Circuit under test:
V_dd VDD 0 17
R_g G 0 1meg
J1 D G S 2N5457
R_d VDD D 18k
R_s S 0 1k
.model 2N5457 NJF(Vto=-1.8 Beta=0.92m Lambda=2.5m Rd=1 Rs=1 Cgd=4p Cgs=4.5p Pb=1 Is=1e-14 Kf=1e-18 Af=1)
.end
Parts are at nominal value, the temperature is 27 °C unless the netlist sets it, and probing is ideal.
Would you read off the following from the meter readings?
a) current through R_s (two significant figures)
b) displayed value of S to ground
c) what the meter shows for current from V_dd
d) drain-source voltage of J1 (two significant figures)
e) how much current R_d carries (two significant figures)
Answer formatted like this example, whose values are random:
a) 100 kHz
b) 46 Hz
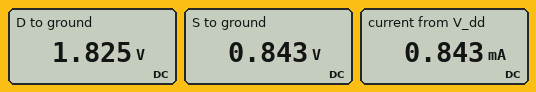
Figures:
a) 840 µA
b) 0.843 V
c) 0.843 mA
d) 980 mV
e) 840 µA
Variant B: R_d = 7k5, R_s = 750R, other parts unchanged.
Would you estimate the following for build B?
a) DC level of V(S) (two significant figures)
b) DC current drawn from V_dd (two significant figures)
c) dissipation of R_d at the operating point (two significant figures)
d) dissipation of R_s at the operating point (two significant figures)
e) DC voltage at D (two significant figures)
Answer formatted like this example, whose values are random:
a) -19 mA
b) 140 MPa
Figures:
a) 760 mV
b) 1.0 mA
c) 7.7 mW
d) 770 µW
e) 9.4 V
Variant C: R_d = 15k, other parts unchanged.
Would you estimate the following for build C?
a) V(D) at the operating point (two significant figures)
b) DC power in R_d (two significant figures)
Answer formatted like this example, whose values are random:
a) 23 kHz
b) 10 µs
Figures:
a) 4.3 V
b) 11 mW
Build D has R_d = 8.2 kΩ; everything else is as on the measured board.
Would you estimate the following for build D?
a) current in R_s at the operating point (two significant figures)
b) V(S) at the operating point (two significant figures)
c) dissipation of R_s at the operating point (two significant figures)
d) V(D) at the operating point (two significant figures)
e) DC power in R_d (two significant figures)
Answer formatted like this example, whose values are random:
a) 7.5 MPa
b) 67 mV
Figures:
a) 850 µA
b) 850 mV
c) 720 µW
d) 10 V
e) 5.9 mW
